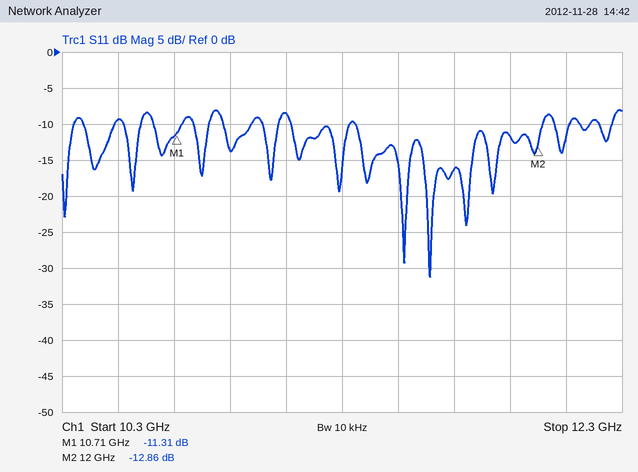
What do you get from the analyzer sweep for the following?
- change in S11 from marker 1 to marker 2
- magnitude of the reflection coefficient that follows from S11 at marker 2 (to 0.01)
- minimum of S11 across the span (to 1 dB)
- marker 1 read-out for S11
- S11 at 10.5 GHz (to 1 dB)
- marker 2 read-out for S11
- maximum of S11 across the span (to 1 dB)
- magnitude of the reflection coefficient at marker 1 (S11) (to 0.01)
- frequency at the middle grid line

-1.55 dB
0.23
-31 dB
-11.31 dB
-9 dB
-12.86 dB
-8 dB
0.27
11.3 GHz
